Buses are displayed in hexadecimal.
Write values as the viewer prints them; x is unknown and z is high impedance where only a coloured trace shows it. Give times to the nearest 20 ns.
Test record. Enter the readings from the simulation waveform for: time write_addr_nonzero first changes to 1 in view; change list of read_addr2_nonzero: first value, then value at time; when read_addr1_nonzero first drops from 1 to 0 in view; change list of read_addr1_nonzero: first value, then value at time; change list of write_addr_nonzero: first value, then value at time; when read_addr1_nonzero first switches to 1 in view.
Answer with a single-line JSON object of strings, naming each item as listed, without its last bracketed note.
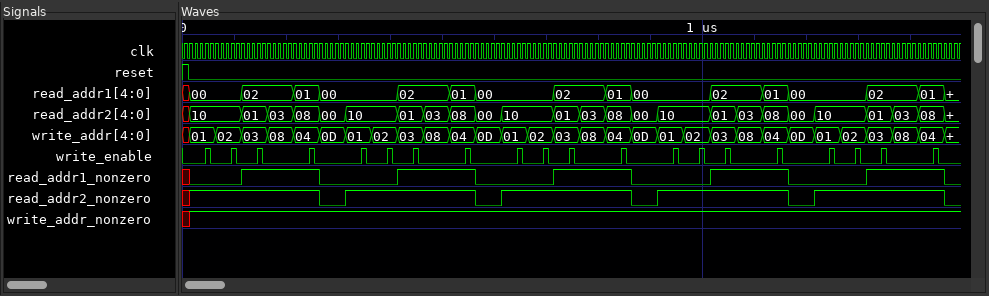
{"time write_addr_nonzero first changes to 1 in view": "20 ns", "change list of read_addr2_nonzero: first value, then value at time": "x, 1 at 20 ns, 0 at 260 ns, 1 at 320 ns, 0 at 560 ns, 1 at 620 ns, 0 at 860 ns, 1 at 920 ns, 0 at 1160 ns, 1 at 1220 ns, 0 at 1460 ns", "when read_addr1_nonzero first drops from 1 to 0 in view": "260 ns", "change list of read_addr1_nonzero: first value, then value at time": "x, 0 at 20 ns, 1 at 120 ns, 0 at 260 ns, 1 at 420 ns, 0 at 560 ns, 1 at 720 ns, 0 at 860 ns, 1 at 1020 ns, 0 at 1160 ns, 1 at 1320 ns, 0 at 1460 ns", "change list of write_addr_nonzero: first value, then value at time": "x, 1 at 20 ns", "when read_addr1_nonzero first switches to 1 in view": "120 ns"}
